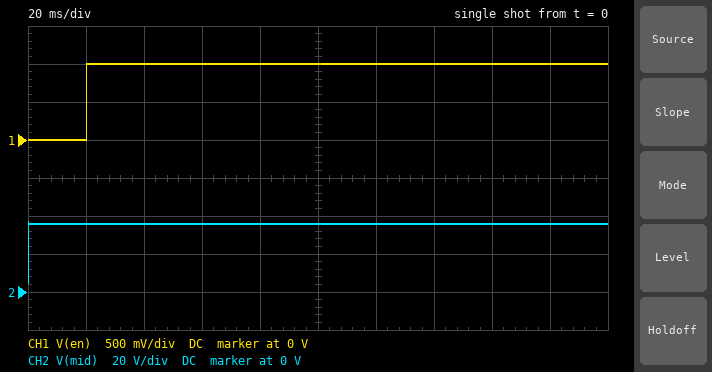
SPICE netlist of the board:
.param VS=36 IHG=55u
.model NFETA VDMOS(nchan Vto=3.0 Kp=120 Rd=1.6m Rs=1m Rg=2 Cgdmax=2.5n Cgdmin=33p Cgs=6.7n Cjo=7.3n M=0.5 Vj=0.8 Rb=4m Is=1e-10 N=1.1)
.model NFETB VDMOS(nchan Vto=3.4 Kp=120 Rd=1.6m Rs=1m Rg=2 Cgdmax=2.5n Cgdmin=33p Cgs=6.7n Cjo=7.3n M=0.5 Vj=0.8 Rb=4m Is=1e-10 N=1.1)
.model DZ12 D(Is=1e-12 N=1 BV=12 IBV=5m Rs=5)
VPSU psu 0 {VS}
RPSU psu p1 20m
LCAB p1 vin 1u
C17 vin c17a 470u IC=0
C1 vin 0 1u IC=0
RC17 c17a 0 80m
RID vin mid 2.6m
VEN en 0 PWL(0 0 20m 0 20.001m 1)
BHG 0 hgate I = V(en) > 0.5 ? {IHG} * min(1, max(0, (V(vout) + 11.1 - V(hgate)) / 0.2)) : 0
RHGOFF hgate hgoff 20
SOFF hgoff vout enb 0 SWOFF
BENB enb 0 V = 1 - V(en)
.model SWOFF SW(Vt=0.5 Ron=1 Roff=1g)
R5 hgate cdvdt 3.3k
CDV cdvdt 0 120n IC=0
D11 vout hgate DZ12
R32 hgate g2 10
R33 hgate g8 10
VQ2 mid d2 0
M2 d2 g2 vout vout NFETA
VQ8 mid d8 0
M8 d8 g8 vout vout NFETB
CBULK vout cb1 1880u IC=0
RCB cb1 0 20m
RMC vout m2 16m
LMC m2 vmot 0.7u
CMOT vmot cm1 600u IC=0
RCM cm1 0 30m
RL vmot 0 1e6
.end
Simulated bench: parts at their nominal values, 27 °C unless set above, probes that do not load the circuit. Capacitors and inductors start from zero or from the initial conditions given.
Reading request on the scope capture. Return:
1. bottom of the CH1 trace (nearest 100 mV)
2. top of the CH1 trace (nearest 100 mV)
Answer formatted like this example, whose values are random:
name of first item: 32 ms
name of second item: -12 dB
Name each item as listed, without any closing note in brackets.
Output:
bottom of the CH1 trace: 0 V
top of the CH1 trace: 1.0 V
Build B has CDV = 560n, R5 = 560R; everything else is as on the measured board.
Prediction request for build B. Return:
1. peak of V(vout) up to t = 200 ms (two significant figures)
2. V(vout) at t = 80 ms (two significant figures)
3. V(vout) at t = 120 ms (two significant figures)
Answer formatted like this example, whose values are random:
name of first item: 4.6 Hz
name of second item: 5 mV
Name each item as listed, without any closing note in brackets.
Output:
peak of V(vout) up to t = 200 ms: 15 V
V(vout) at t = 80 ms: 2.9 V
V(vout) at t = 120 ms: 6.8 V
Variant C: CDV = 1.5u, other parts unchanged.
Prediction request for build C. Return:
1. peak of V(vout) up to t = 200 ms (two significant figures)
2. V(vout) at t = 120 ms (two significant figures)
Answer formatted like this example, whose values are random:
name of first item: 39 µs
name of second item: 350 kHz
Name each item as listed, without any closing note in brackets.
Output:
peak of V(vout) up to t = 200 ms: 3.8 V
V(vout) at t = 120 ms: 900 mV
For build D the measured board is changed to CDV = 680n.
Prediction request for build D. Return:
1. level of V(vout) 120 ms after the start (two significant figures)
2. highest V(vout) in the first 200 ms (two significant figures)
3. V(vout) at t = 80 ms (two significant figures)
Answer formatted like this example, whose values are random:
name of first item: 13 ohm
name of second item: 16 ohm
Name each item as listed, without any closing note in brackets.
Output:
level of V(vout) 120 ms after the start: 5.2 V
highest V(vout) in the first 200 ms: 12 V
V(vout) at t = 80 ms: 2.0 V
